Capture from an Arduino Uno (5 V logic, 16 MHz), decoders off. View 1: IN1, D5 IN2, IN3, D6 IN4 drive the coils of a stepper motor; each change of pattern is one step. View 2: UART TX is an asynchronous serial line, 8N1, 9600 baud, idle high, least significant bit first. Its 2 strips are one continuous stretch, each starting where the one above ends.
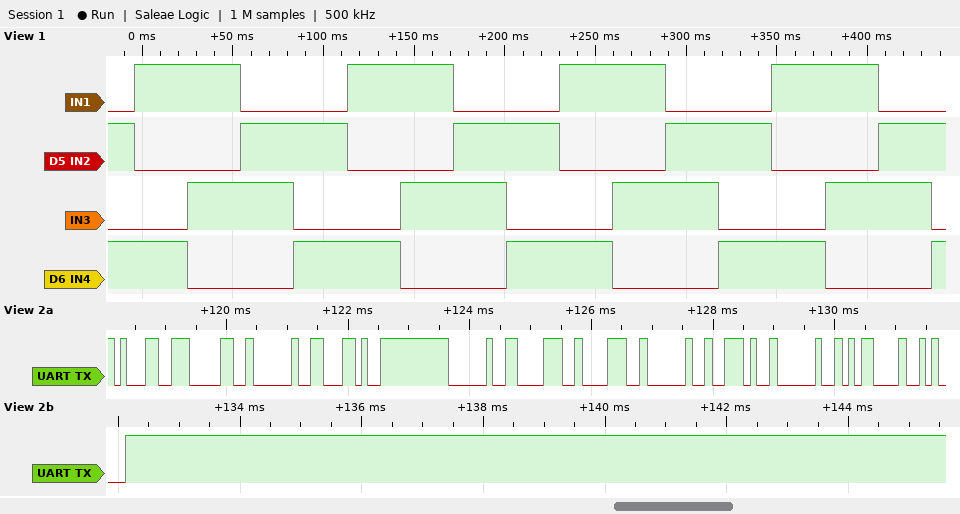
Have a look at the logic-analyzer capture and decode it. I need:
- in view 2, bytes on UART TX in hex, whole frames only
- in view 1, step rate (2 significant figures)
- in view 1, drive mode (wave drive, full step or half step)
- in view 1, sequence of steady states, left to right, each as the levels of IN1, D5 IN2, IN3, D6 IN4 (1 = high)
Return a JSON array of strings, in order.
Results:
["31 30 20 2C 20 38 38 20 2E 20 0D 0A", "34 steps/s", "full step", "0101 1001 1010 0110 0101 1001 1010 0110 0101 1001 1010 0110 0101 1001 1010 0110 0101"]
